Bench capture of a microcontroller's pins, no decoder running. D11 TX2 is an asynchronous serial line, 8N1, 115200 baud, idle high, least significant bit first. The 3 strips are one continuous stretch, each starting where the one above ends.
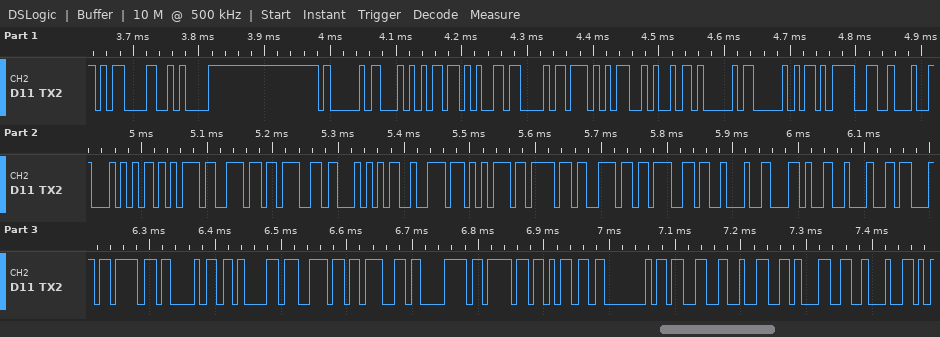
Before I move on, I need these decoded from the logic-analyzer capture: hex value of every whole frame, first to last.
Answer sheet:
0D 0A 41 54 2B 43 57 4A 41 50 3D 22 54 75 6E 67 54 72 75 6F 6E 67 22 2C 22 63 6F 68 61 6E 67 78 6F 6D 40 33 32 31 22
